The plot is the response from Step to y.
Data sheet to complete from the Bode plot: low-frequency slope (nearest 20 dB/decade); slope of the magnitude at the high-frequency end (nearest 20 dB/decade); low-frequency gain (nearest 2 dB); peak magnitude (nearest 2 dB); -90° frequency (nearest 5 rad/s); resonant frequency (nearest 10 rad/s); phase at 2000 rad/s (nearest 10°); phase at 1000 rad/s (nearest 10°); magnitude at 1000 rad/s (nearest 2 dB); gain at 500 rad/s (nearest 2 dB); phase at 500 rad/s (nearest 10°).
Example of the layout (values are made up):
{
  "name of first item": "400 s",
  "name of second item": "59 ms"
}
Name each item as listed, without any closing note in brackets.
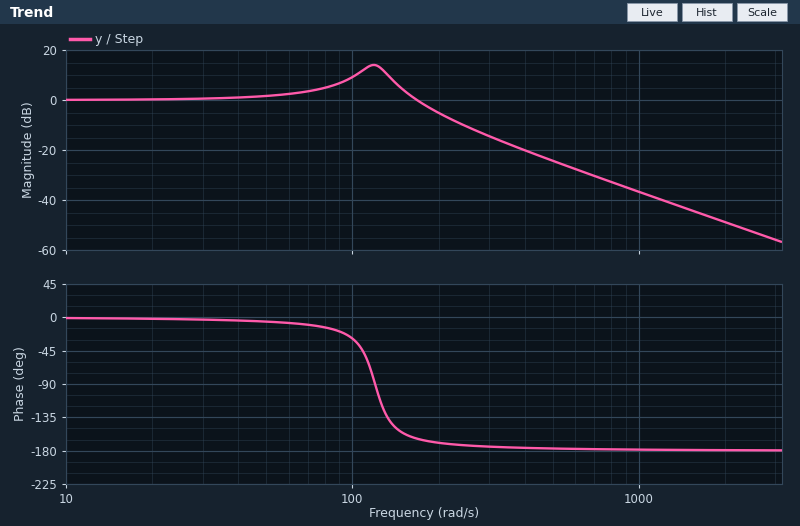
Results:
{
  "low-frequency slope": "0 dB/decade",
  "slope of the magnitude at the high-frequency end": "-40 dB/decade",
  "low-frequency gain": "0 dB",
  "peak magnitude": "14 dB",
  "-90° frequency": "120 rad/s",
  "resonant frequency": "120 rad/s",
  "phase at 2000 rad/s": "-180°",
  "phase at 1000 rad/s": "-180°",
  "magnitude at 1000 rad/s": "-36 dB",
  "gain at 500 rad/s": "-24 dB",
  "phase at 500 rad/s": "-180°"
}
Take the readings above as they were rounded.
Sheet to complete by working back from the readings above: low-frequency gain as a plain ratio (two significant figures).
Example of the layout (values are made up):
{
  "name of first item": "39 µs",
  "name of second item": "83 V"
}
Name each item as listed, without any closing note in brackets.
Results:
{
  "low-frequency gain as a plain ratio": "1.0"
}
